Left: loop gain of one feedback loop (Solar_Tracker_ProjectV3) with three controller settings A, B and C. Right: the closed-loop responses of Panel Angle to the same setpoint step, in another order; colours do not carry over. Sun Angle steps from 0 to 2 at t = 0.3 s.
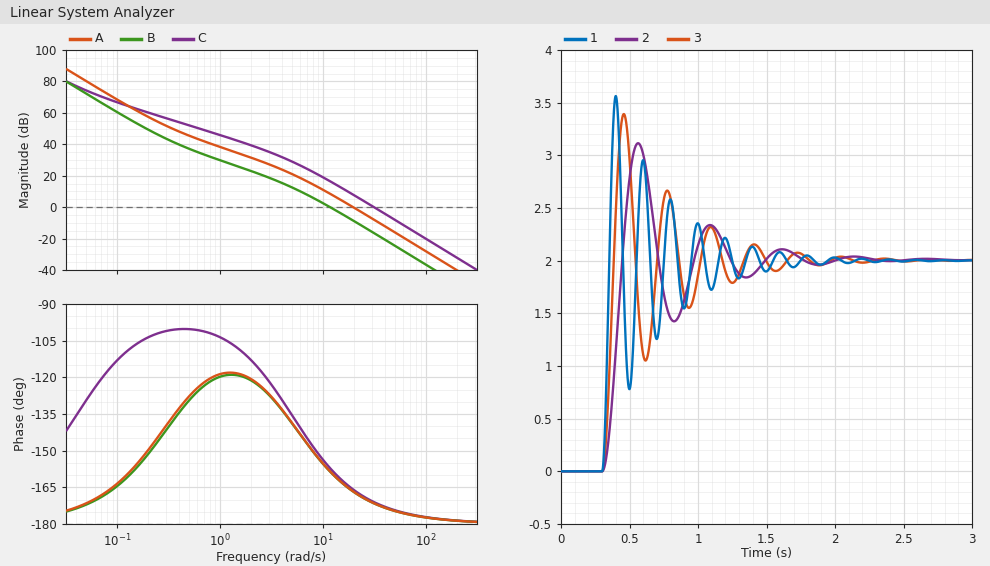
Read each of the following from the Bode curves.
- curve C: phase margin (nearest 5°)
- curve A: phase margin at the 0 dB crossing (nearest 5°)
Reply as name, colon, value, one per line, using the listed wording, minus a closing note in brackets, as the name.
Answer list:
curve C: phase margin: 10°
curve A: phase margin at the 0 dB crossing: 15°
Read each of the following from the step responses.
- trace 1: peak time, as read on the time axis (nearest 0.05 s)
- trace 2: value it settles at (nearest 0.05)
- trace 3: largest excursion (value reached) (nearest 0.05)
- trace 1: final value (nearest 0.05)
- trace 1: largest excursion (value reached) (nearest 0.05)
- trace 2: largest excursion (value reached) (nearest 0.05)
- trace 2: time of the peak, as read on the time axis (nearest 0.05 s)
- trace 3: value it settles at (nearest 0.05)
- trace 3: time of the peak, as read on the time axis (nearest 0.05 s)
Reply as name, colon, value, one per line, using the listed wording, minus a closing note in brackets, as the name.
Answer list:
trace 1: peak time, as read on the time axis: 0.40 s
trace 2: value it settles at: 2.00
trace 3: largest excursion (value reached): 3.40
trace 1: final value: 2.00
trace 1: largest excursion (value reached): 3.55
trace 2: largest excursion (value reached): 3.10
trace 2: time of the peak, as read on the time axis: 0.55 s
trace 3: value it settles at: 2.00
trace 3: time of the peak, as read on the time axis: 0.45 s
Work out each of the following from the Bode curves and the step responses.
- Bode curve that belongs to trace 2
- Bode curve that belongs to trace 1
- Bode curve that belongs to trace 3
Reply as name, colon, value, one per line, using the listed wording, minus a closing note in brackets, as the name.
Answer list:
Bode curve that belongs to trace 2: B
Bode curve that belongs to trace 1: C
Bode curve that belongs to trace 3: A
